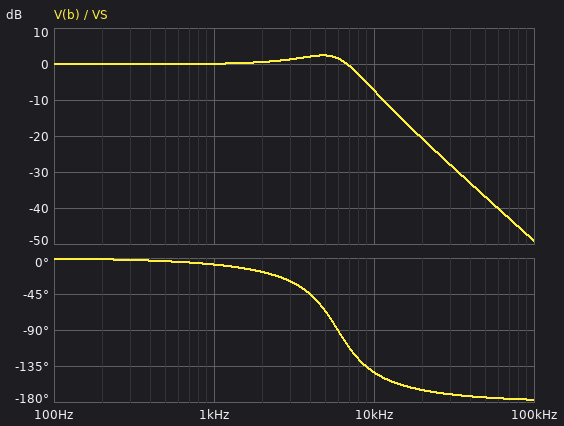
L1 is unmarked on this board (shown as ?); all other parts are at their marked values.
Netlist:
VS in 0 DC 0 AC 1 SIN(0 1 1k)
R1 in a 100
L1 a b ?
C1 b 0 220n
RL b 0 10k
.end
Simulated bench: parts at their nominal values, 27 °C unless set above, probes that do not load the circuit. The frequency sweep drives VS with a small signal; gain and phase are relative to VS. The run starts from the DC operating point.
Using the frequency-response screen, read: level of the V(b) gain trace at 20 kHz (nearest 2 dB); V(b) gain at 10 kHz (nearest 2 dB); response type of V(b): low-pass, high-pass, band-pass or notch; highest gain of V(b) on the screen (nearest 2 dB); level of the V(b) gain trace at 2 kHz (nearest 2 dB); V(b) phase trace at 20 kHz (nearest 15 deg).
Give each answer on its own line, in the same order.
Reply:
-20 dB
-8 dB
low-pass
2 dB
0 dB
-165 deg
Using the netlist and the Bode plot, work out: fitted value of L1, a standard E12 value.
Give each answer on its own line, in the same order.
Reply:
3.3 mH
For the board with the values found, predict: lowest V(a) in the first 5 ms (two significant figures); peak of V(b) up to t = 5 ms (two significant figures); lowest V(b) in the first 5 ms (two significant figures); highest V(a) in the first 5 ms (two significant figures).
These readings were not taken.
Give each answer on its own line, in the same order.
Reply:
-980 mV
1.0 V
-1.0 V
980 mV
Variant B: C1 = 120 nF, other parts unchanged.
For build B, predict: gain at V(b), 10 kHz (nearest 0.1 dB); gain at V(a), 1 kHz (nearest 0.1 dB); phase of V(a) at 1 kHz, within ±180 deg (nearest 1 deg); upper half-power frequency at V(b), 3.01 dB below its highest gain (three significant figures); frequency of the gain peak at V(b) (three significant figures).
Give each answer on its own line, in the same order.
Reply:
0.4 dB
-0.1 dB
-4 deg
9.50 kHz
7.23 kHz
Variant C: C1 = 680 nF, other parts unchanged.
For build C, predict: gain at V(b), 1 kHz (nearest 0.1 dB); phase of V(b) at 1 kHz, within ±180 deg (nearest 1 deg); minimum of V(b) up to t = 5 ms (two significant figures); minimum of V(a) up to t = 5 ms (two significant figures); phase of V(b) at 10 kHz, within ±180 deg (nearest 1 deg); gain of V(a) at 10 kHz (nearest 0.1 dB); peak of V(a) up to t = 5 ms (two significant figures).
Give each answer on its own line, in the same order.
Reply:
-0.1 dB
-25 deg
-980 mV
-900 mV
-151 deg
-1.1 dB
900 mV
